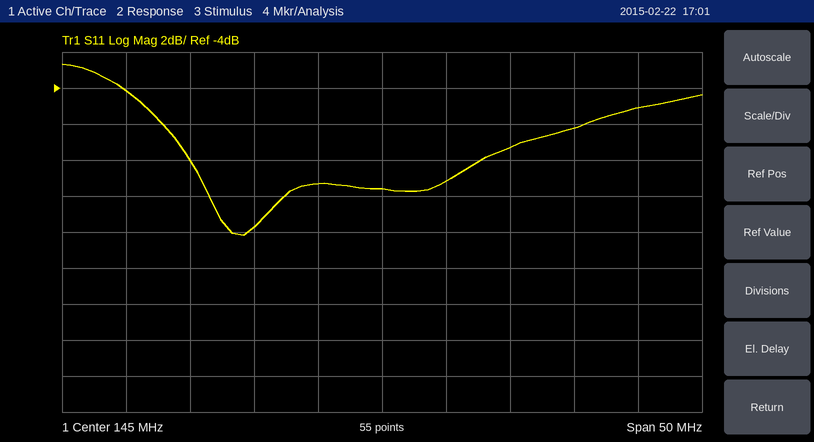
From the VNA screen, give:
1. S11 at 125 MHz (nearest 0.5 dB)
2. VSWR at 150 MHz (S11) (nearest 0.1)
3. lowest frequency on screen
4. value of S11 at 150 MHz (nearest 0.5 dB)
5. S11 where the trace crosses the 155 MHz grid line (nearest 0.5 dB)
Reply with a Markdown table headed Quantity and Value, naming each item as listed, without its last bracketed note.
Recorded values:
| Quantity | Value |
|---|---|
| S11 at 125 MHz | -4.0 dB |
| VSWR at 150 MHz (S11) | 2.1 |
| lowest frequency on screen | 120 MHz |
| value of S11 at 150 MHz | -9.0 dB |
| S11 where the trace crosses the 155 MHz grid line | -7.5 dB |
